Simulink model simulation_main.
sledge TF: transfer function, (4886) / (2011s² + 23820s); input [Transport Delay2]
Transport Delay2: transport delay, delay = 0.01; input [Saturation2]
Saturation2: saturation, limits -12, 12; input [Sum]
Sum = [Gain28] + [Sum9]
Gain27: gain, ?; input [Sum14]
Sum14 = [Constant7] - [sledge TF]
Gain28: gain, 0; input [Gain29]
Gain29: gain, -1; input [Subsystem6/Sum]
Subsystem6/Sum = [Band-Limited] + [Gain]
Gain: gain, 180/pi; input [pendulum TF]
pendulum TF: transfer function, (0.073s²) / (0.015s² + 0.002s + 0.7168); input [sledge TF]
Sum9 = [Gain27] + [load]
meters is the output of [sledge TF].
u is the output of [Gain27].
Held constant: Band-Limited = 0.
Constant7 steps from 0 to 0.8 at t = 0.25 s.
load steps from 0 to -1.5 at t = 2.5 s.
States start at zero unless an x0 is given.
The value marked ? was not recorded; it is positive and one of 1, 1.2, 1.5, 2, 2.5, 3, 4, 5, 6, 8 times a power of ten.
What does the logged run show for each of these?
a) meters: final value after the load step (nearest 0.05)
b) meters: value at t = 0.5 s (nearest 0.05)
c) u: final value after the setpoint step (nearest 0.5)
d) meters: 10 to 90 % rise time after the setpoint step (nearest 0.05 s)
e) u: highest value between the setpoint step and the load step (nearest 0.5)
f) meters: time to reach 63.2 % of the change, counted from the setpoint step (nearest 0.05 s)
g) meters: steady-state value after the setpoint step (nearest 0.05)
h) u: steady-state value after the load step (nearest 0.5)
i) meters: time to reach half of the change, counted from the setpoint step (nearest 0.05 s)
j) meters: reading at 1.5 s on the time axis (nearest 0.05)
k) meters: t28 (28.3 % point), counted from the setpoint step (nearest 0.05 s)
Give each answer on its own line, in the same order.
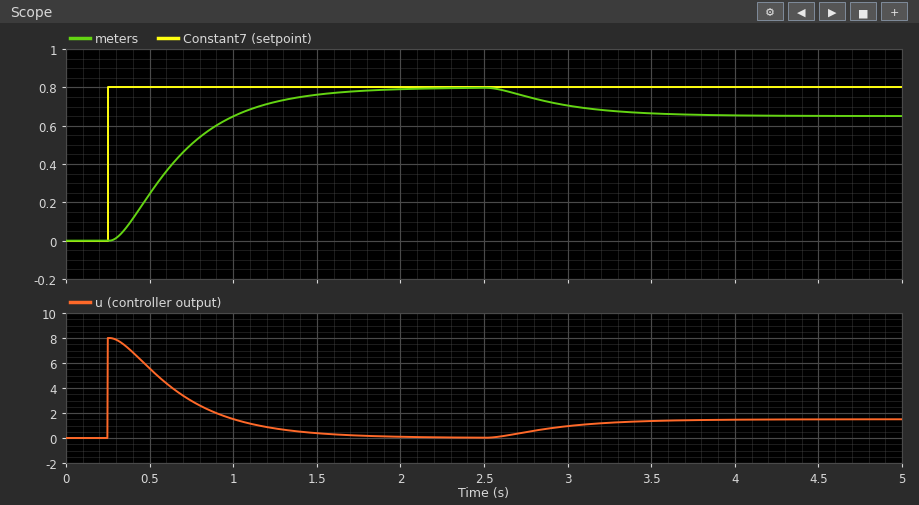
0.65
0.25
0.0
0.85 s
8.0
0.50 s
0.80
1.5
0.40 s
0.75
0.25 s
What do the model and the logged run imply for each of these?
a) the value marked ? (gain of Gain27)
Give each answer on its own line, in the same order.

10
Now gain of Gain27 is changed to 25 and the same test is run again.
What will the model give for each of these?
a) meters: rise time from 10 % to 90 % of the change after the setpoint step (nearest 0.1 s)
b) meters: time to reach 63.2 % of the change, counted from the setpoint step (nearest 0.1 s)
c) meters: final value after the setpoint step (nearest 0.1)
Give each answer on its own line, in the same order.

0.3 s
0.3 s
0.8
